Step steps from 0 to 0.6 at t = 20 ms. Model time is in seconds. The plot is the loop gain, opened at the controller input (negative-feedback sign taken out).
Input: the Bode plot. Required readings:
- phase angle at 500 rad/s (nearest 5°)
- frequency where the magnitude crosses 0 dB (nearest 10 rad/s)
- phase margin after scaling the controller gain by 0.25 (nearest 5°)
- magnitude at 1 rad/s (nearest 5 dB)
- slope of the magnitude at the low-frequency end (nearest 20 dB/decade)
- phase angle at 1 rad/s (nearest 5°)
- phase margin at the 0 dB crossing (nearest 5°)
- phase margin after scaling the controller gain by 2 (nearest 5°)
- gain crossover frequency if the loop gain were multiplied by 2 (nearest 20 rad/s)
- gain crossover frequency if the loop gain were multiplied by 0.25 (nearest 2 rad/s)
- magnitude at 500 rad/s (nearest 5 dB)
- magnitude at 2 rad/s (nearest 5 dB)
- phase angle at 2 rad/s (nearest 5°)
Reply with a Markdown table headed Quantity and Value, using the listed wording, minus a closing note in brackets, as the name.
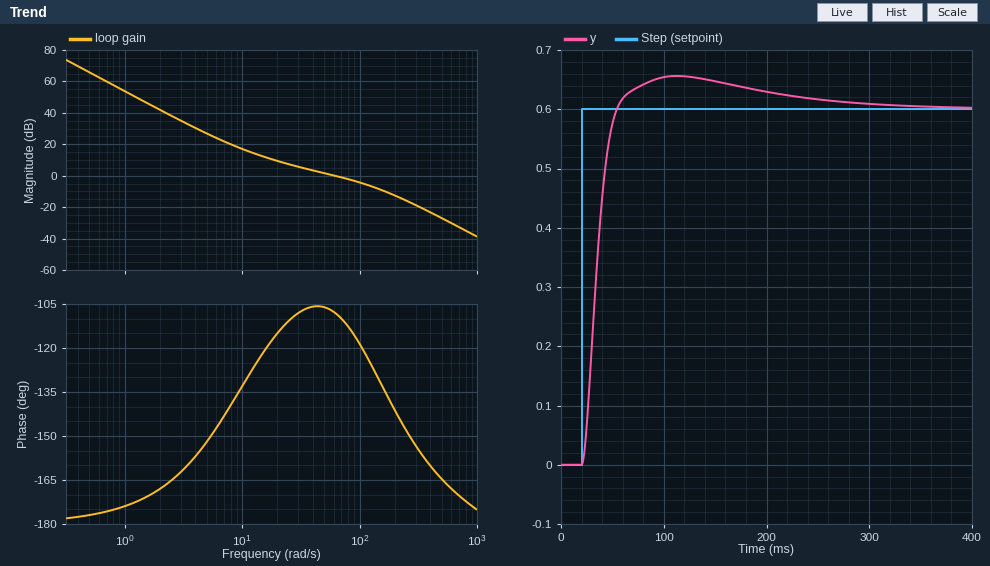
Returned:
| Quantity | Value |
|---|---|
| phase angle at 500 rad/s | -165° |
| frequency where the magnitude crosses 0 dB | 60 rad/s |
| phase margin after scaling the controller gain by 0.25 | 60° |
| magnitude at 1 rad/s | 55 dB |
| slope of the magnitude at the low-frequency end | -40 dB/decade |
| phase angle at 1 rad/s | -175° |
| phase margin at the 0 dB crossing | 70° |
| phase margin after scaling the controller gain by 2 | 55° |
| gain crossover frequency if the loop gain were multiplied by 2 | 120 rad/s |
| gain crossover frequency if the loop gain were multiplied by 0.25 | 16 rad/s |
| magnitude at 500 rad/s | -25 dB |
| magnitude at 2 rad/s | 40 dB |
| phase angle at 2 rad/s | -170° |
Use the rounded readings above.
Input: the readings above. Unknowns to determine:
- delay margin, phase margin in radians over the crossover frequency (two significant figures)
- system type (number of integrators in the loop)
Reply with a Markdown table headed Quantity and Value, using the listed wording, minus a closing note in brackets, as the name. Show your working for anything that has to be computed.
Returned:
| Quantity | Value |
|---|---|
| delay margin, phase margin in radians over the crossover frequency | 70 × π / 180 / 60 = 0.020 s |
| system type | 2 |
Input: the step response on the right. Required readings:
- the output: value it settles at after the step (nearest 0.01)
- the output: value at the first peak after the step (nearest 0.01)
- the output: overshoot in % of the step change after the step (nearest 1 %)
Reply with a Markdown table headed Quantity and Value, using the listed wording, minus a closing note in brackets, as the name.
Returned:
| Quantity | Value |
|---|---|
| the output: value it settles at after the step | 0.60 |
| the output: value at the first peak after the step | 0.66 |
| the output: overshoot in % of the step change after the step | 9 % |
